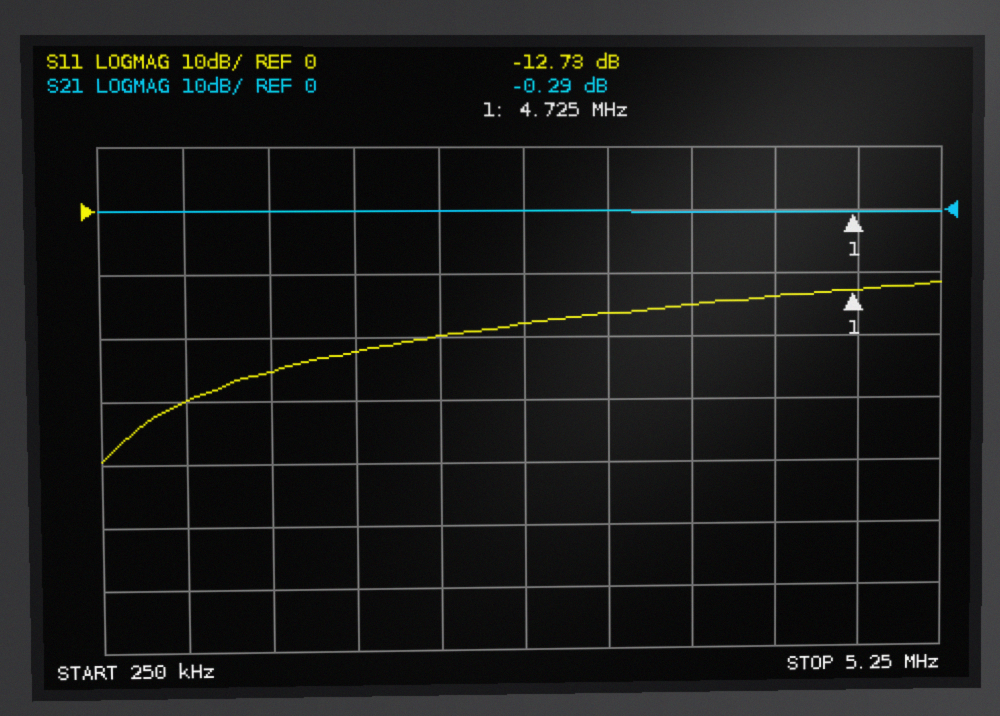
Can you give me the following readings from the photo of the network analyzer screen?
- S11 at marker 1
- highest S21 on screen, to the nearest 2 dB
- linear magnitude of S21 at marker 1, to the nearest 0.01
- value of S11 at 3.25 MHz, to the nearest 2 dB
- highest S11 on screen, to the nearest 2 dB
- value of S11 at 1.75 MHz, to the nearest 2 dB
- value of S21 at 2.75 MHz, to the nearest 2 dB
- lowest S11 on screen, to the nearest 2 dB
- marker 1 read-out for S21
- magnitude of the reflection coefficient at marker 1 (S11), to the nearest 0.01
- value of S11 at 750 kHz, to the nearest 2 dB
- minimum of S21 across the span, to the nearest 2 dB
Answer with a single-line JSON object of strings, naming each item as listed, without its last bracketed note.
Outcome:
{"S11 at marker 1": "-12.73 dB", "highest S21 on screen, to the nearest 2 dB": "0 dB", "linear magnitude of S21 at marker 1, to the nearest 0.01": "0.97", "value of S11 at 3.25 MHz, to the nearest 2 dB": "-16 dB", "highest S11 on screen, to the nearest 2 dB": "-12 dB", "value of S11 at 1.75 MHz, to the nearest 2 dB": "-22 dB", "value of S21 at 2.75 MHz, to the nearest 2 dB": "0 dB", "lowest S11 on screen, to the nearest 2 dB": "-40 dB", "marker 1 read-out for S21": "-0.29 dB", "magnitude of the reflection coefficient at marker 1 (S11), to the nearest 0.01": "0.23", "value of S11 at 750 kHz, to the nearest 2 dB": "-30 dB", "minimum of S21 across the span, to the nearest 2 dB": "0 dB"}
